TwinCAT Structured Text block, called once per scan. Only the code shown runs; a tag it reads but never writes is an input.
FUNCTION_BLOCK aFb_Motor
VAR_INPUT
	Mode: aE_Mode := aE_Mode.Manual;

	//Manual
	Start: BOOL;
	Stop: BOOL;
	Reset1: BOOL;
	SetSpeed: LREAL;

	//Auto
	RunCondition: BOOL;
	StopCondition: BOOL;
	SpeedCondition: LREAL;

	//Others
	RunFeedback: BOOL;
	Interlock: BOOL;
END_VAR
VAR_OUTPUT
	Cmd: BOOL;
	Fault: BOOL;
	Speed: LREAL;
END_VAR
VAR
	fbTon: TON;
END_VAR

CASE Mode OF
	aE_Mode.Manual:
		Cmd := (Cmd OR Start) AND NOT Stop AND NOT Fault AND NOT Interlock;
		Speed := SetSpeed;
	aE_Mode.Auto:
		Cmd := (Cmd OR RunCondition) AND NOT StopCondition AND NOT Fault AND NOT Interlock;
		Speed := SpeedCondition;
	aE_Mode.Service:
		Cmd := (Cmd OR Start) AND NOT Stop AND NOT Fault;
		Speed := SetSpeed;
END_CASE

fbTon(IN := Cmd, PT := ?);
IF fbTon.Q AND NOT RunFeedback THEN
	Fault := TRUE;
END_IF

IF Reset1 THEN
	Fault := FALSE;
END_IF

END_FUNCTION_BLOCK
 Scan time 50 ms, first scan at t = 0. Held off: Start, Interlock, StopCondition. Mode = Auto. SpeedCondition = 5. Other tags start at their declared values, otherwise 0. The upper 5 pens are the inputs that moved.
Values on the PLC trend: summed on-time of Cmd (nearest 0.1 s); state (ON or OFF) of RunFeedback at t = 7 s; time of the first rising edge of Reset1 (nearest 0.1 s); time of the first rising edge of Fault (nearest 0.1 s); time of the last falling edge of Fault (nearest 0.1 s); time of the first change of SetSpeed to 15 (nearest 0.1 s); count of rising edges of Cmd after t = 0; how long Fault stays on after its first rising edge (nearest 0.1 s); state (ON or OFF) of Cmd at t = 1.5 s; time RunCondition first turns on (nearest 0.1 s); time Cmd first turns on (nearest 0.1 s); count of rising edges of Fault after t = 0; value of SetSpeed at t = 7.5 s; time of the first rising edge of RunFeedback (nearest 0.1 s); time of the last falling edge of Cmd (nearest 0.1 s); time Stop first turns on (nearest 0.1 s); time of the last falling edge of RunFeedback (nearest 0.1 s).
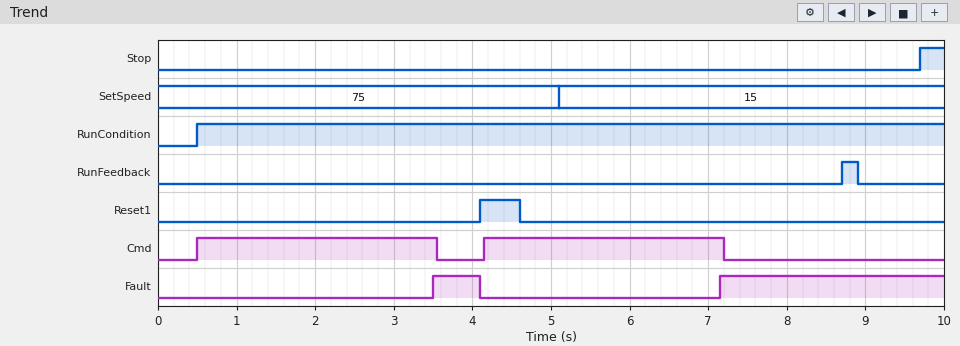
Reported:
6.1 s
OFF
4.1 s
3.5 s
4.1 s
5.1 s
2
0.6 s
ON
0.5 s
0.5 s
2
15
8.7 s
7.2 s
9.7 s
8.9 s
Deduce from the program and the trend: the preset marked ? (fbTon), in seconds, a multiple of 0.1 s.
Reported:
3.0 s
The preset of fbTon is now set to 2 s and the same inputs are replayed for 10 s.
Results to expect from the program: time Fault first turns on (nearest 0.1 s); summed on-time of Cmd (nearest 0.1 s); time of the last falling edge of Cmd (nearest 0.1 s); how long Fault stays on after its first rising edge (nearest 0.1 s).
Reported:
2.5 s
4.1 s
6.2 s
1.6 s
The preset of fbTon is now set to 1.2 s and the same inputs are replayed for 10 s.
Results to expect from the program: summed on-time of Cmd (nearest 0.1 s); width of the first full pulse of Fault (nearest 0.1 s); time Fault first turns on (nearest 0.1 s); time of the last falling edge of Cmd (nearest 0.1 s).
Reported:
2.5 s
2.4 s
1.7 s
5.4 s
